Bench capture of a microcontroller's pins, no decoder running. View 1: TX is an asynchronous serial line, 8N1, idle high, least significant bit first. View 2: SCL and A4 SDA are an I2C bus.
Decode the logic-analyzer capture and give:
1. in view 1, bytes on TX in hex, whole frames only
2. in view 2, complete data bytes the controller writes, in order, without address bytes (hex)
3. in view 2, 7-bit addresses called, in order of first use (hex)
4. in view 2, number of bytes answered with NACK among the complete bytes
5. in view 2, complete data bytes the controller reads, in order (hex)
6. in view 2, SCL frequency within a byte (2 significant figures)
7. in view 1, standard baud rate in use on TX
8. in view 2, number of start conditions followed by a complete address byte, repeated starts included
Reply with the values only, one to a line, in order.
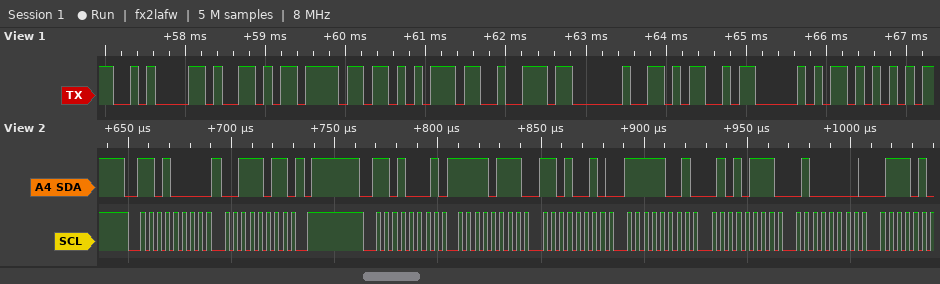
0A 59 6F 75 72 20 4D 50 55
3B
0x68
0
F7 D2 F9 57 40
250 kHz
9600 baud
2
